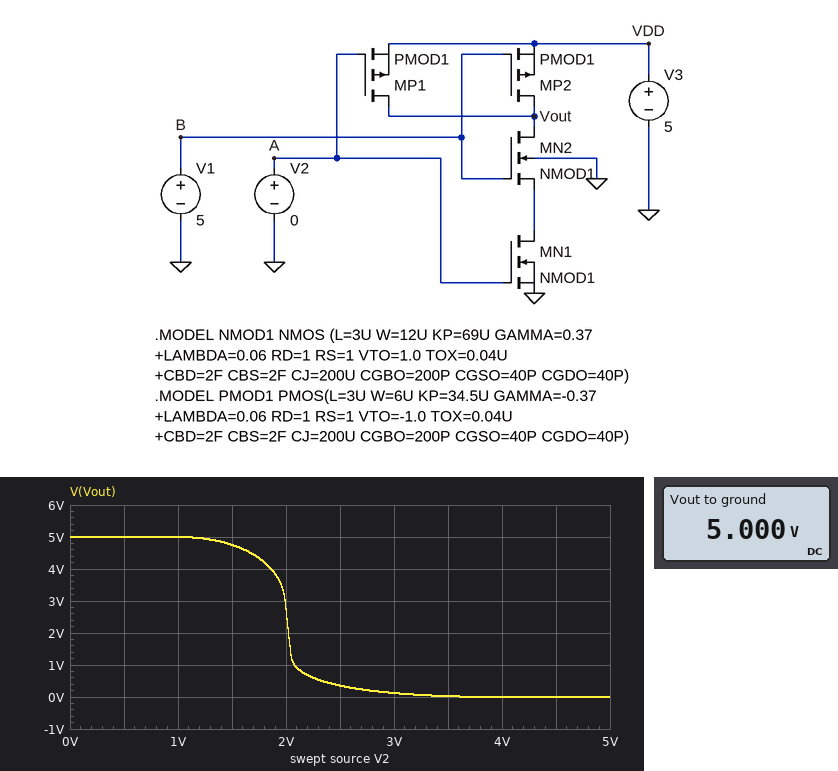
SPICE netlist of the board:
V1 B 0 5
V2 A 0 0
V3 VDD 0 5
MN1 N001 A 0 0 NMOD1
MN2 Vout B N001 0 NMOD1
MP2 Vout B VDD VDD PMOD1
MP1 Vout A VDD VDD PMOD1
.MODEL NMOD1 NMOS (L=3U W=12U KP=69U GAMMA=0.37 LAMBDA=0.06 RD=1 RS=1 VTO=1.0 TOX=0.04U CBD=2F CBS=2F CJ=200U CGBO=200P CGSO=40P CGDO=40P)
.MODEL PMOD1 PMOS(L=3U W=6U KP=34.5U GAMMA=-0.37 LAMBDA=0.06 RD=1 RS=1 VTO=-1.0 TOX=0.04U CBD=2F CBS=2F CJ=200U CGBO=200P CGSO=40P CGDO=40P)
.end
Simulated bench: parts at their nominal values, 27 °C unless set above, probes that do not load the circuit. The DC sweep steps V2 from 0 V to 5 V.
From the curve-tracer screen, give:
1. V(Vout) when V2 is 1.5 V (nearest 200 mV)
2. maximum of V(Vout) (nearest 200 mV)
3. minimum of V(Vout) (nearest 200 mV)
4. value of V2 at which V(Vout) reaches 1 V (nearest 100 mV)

4.8 V
5.0 V
0 V
2.1 V
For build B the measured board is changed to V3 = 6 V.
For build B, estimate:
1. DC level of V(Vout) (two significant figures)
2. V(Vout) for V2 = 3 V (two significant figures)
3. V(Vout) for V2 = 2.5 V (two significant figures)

6.0 V
550 mV
1.3 V
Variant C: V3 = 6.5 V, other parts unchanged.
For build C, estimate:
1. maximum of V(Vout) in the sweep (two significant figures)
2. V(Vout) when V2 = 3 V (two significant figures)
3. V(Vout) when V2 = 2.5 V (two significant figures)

6.5 V
960 mV
4.1 V
